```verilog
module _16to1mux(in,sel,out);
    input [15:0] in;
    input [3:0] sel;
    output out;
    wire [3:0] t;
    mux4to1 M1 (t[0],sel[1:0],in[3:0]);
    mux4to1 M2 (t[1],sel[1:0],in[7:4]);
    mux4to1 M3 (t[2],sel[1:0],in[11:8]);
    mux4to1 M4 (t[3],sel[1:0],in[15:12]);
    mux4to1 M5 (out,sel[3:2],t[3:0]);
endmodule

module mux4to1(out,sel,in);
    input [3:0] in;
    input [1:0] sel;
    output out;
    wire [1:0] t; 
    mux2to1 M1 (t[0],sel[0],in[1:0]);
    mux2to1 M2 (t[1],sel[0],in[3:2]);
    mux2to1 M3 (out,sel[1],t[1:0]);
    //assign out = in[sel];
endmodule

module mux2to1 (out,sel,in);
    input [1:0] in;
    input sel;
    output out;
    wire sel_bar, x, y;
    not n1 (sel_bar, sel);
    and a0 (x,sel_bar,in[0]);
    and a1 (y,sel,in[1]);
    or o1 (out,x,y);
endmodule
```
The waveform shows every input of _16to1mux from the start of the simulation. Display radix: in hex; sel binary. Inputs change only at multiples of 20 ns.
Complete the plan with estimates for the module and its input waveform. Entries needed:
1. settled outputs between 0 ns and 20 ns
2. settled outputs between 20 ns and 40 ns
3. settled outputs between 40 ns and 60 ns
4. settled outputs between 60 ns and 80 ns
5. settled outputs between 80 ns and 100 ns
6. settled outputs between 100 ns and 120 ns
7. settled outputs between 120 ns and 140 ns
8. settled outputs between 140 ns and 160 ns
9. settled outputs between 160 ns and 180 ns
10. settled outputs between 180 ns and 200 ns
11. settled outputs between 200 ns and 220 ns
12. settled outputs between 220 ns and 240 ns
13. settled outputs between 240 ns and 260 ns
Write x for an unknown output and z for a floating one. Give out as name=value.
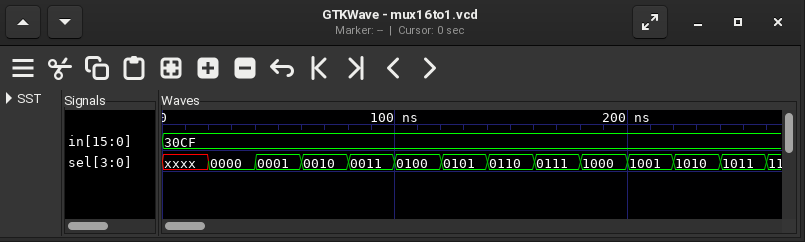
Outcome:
out=x
out=1
out=1
out=1
out=1
out=0
out=0
out=1
out=1
out=0
out=0
out=0
out=0
